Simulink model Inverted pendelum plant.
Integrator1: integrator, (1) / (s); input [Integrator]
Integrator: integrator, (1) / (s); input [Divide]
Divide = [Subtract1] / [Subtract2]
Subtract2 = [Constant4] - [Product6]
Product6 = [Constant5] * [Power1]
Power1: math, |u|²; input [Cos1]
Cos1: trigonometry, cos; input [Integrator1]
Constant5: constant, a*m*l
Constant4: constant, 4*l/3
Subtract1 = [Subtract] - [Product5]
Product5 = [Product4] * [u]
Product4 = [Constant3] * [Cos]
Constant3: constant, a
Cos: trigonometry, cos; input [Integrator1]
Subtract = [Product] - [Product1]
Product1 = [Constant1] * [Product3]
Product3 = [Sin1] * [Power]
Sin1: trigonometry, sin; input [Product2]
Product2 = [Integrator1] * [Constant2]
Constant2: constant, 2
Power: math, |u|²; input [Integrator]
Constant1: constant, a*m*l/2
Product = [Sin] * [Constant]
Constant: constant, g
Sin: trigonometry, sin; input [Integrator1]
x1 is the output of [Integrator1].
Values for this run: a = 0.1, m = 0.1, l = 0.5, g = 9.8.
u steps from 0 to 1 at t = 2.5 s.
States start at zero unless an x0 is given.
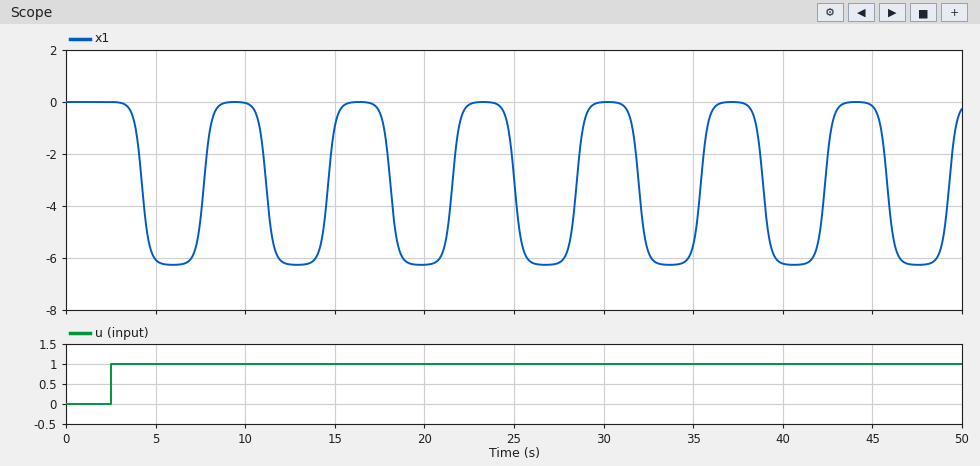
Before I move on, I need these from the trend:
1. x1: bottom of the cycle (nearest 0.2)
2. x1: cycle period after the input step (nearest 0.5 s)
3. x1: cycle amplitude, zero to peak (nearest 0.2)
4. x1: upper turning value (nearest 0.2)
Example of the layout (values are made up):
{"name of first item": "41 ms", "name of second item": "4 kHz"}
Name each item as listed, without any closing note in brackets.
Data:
{"x1: bottom of the cycle": "-6.2", "x1: cycle period after the input step": "7.0 s", "x1: cycle amplitude, zero to peak": "3.2", "x1: upper turning value": "0.0"}
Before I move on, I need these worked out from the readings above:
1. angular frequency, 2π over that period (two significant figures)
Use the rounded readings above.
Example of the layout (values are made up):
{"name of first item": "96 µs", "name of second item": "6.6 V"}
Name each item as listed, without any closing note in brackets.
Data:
{"angular frequency, 2π over that period": "0.90 rad/s"}
